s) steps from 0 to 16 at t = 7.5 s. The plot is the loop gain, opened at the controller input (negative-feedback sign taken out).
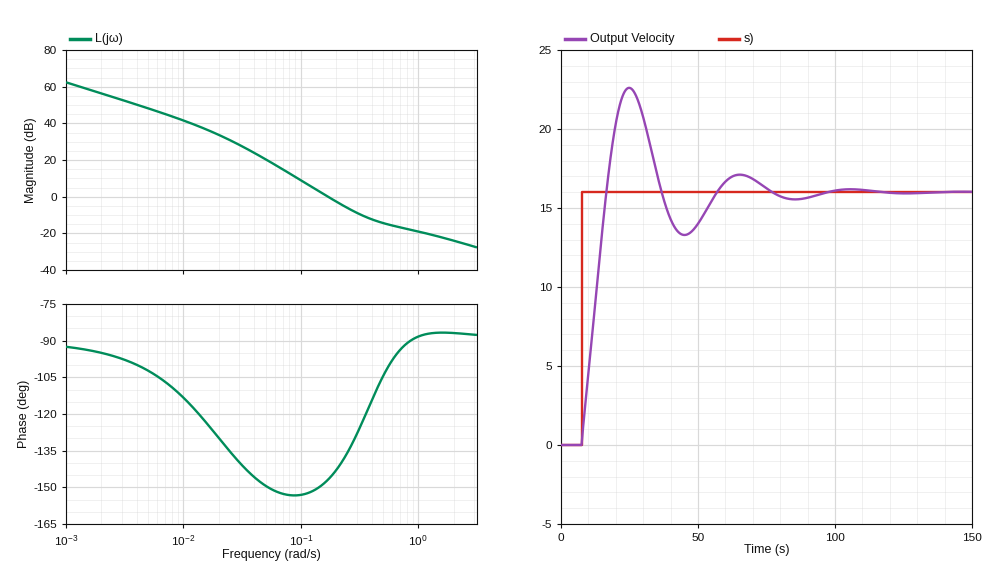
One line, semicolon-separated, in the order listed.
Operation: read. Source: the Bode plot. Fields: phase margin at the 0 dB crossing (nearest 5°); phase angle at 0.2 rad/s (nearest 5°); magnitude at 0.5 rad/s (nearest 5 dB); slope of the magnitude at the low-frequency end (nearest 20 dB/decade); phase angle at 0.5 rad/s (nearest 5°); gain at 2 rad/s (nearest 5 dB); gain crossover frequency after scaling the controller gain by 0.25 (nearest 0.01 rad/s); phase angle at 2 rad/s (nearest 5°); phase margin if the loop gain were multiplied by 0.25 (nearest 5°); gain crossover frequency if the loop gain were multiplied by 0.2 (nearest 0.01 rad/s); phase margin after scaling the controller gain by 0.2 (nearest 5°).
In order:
35°; -145°; -15 dB; -20 dB/decade; -105°; -25 dB; 0.08 rad/s; -85°; 25°; 0.07 rad/s; 25°
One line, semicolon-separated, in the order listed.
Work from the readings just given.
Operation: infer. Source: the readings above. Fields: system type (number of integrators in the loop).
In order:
1
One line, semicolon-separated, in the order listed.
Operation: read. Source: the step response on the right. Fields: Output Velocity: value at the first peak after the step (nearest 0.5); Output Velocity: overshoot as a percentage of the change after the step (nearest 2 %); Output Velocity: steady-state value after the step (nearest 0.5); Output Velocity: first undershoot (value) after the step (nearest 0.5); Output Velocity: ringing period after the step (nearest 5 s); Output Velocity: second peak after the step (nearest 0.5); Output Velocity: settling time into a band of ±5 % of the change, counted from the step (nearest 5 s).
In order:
22.5; 42 %; 16.0; 13.5; 40 s; 17.0; 65 s
